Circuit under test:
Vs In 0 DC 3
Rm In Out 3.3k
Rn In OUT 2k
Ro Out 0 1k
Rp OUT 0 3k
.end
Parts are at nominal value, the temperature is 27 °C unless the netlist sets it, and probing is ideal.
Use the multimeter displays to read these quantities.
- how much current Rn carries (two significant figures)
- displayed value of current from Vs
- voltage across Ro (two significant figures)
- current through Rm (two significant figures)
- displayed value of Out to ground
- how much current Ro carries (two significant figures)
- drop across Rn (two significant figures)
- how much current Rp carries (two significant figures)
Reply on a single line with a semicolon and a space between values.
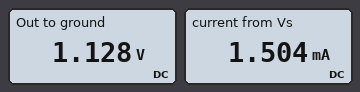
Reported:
940 µA; 1.504 mA; 1.1 V; 570 µA; 1.128 V; 1.1 mA; 1.9 V; 380 µA
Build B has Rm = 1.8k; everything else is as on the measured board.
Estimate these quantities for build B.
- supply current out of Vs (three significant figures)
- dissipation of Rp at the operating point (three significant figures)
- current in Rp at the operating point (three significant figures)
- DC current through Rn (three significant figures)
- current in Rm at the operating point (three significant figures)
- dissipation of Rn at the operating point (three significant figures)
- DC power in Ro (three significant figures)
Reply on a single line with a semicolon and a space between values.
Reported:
1.77 mA; 586 µW; 442 µA; 837 µA; 930 µA; 1.40 mW; 1.76 mW
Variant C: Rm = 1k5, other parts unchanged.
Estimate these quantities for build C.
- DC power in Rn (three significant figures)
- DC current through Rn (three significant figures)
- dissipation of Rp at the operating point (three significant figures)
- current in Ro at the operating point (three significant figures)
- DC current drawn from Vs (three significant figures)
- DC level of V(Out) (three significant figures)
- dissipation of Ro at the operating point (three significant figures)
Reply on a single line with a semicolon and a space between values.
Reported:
1.28 mW; 800 µA; 653 µW; 1.40 mA; 1.87 mA; 1.40 V; 1.96 mW
